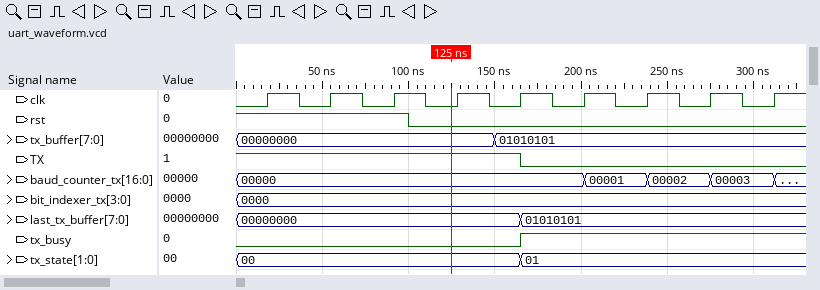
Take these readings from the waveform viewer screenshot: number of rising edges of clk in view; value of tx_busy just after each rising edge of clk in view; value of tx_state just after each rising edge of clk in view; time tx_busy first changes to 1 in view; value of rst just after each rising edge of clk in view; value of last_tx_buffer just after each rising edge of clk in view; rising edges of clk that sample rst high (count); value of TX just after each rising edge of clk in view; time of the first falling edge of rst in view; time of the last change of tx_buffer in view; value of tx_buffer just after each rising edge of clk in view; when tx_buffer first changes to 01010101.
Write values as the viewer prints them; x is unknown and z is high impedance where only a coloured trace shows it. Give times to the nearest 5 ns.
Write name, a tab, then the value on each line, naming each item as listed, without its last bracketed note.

number of rising edges of clk in view	9
value of tx_busy just after each rising edge of clk in view	0 0 0 0 1 1 1 1 1
value of tx_state just after each rising edge of clk in view	00, 00, 00, 00, 01, 01, 01, 01, 01
time tx_busy first changes to 1 in view	165 ns
value of rst just after each rising edge of clk in view	1 1 1 0 0 0 0 0 0
value of last_tx_buffer just after each rising edge of clk in view	00000000, 00000000, 00000000, 00000000, 01010101, 01010101, 01010101, 01010101, 01010101
rising edges of clk that sample rst high	3
value of TX just after each rising edge of clk in view	1 1 1 1 0 0 0 0 0
time of the first falling edge of rst in view	100 ns
time of the last change of tx_buffer in view	150 ns
value of tx_buffer just after each rising edge of clk in view	00000000, 00000000, 00000000, 00000000, 01010101, 01010101, 01010101, 01010101, 01010101
when tx_buffer first changes to 01010101	150 ns
